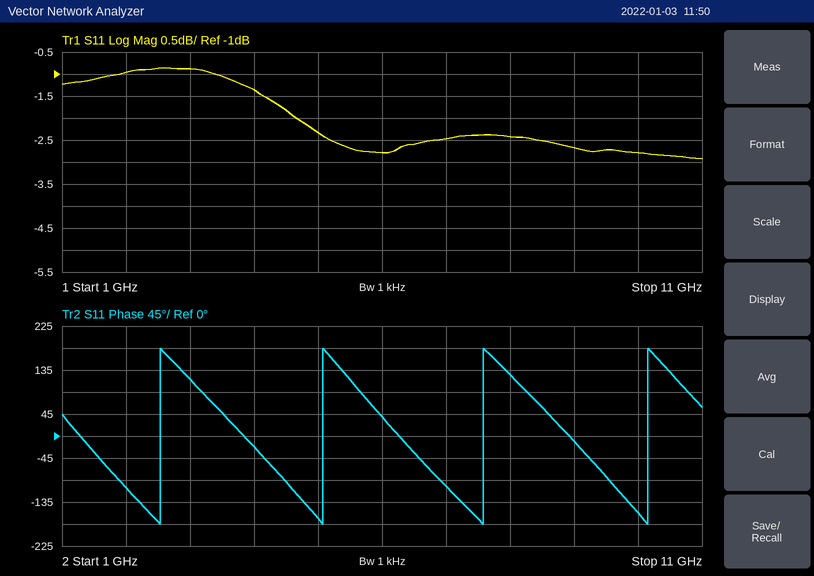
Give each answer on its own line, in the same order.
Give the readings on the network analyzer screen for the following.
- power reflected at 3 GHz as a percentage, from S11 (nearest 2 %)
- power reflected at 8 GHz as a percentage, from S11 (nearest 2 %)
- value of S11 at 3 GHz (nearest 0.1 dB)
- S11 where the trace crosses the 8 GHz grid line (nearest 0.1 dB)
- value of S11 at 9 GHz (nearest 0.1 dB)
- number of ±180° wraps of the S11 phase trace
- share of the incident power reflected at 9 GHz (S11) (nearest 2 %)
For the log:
82 %
58 %
-0.9 dB
-2.4 dB
-2.7 dB
4
54 %
